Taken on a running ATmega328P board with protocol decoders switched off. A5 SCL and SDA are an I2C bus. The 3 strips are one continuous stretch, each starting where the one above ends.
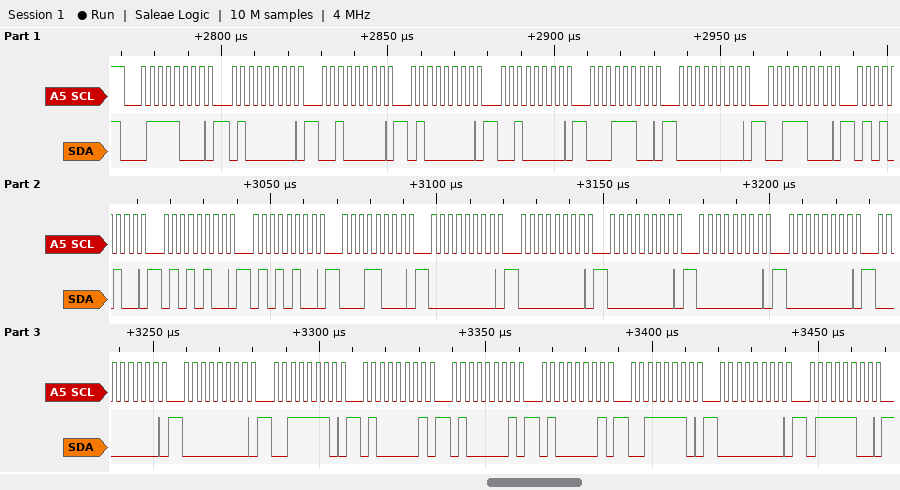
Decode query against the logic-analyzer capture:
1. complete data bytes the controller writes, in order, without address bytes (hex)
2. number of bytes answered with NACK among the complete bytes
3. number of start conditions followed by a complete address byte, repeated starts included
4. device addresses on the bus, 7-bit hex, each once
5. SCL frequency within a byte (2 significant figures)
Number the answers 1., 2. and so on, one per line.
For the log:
1. 40 20 40 20 1C 00 38 54 54 54 18 00 00 00 00 00 00 00 3E 41 41 41 3E 00 7C
2. 0
3. 1
4. 0x3C
5. 400 kHz
